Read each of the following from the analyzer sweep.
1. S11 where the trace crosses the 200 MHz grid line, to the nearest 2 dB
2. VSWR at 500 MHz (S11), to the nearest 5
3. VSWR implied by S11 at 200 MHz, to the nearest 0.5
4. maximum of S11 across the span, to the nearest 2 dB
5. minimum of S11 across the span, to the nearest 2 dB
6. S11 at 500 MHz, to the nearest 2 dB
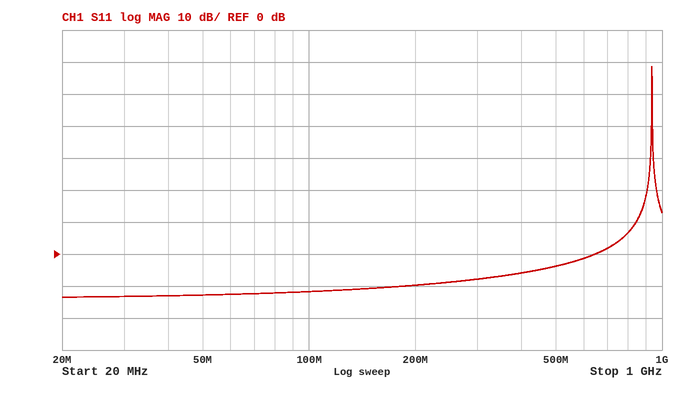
-10 dB
5
2.0
58 dB
-14 dB
-4 dB
